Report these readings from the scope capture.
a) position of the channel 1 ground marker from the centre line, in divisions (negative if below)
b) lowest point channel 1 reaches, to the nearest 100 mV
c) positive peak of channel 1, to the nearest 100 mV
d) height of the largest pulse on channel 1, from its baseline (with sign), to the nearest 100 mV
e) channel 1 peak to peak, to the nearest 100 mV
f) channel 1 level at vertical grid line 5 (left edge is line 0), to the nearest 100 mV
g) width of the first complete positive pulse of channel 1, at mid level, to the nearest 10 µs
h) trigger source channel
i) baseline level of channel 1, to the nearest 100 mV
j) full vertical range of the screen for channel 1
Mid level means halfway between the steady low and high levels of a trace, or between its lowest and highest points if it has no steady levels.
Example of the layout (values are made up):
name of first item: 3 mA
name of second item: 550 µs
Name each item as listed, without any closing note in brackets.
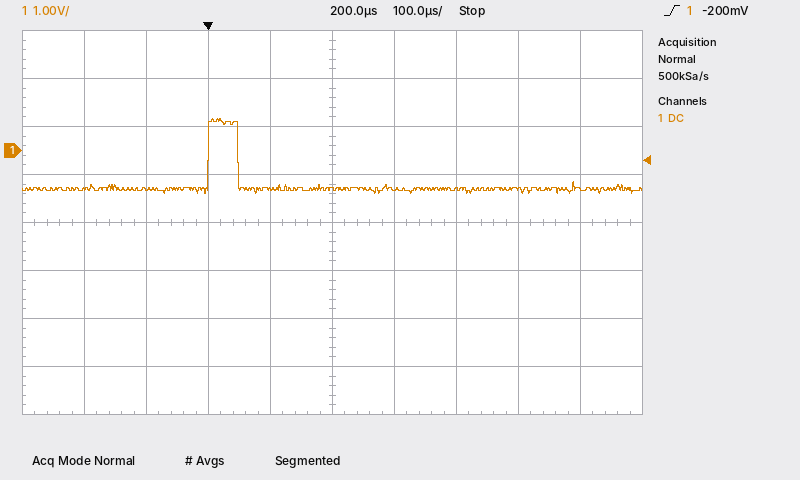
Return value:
position of the channel 1 ground marker from the centre line, in divisions: +1.5 div
lowest point channel 1 reaches, to the nearest 100 mV: -900 mV
positive peak of channel 1, to the nearest 100 mV: 700 mV
height of the largest pulse on channel 1, from its baseline (with sign), to the nearest 100 mV: +1.5 V
channel 1 peak to peak, to the nearest 100 mV: 1.6 V
channel 1 level at vertical grid line 5 (left edge is line 0), to the nearest 100 mV: -800 mV
width of the first complete positive pulse of channel 1, at mid level, to the nearest 10 µs: 50 µs
trigger source channel: channel 1
baseline level of channel 1, to the nearest 100 mV: -800 mV
full vertical range of the screen for channel 1: 8 V
